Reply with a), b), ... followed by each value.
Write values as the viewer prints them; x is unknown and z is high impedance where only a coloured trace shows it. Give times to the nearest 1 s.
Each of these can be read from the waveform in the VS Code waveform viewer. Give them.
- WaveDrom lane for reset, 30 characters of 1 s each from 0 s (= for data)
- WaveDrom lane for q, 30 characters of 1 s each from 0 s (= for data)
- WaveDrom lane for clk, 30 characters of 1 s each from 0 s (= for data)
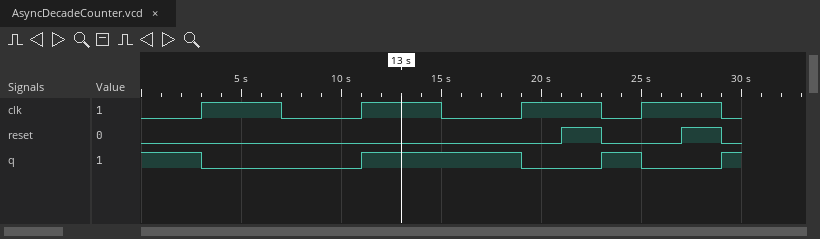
a) {name: 'reset', wave: '0....................1.0...1.0'}
b) {name: 'q', wave: '1..0.......1.......0...1.0...1'}
c) {name: 'clk', wave: '0..1...0...1...0...1...0.1...0'}
